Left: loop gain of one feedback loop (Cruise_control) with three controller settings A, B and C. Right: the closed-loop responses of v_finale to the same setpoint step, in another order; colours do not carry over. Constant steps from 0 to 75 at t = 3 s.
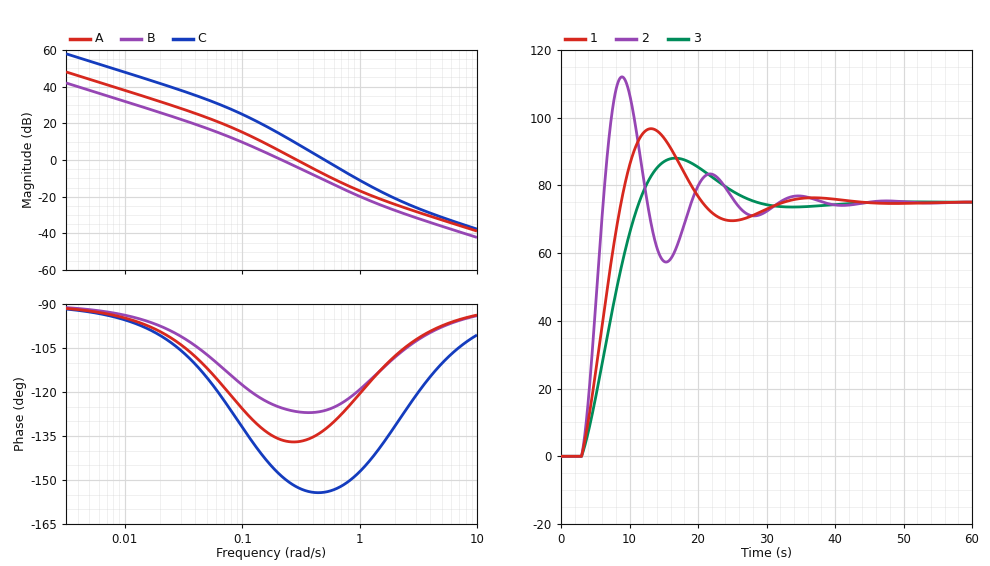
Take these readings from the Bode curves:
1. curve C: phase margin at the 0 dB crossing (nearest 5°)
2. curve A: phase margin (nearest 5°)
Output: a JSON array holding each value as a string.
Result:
["25°", "45°"]
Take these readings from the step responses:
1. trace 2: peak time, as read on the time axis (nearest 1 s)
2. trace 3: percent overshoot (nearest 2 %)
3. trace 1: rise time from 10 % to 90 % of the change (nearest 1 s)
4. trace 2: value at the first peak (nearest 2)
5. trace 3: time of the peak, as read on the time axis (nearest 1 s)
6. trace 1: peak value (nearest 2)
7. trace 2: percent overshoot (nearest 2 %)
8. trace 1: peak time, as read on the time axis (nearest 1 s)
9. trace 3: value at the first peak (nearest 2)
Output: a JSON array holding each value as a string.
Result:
["9 s", "18 %", "4 s", "112", "17 s", "96", "50 %", "13 s", "88"]
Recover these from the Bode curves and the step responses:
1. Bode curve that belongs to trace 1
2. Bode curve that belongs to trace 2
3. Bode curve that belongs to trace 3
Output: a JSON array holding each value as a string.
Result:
["A", "C", "B"]
